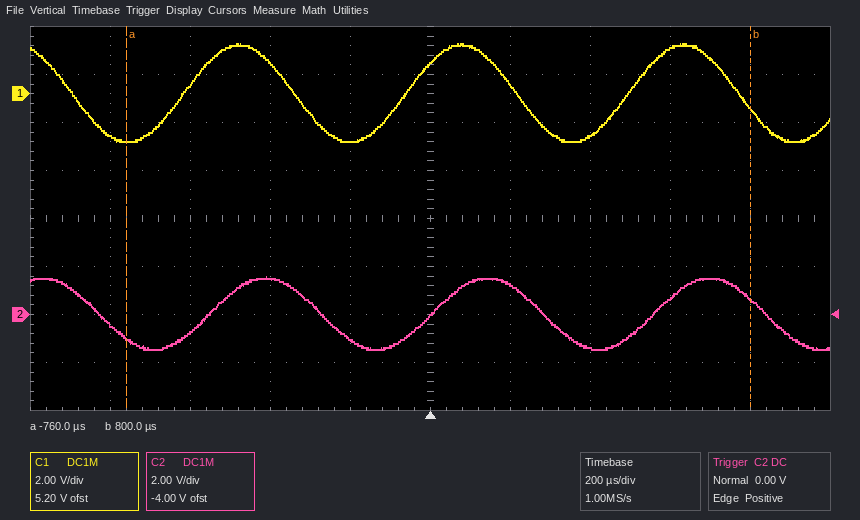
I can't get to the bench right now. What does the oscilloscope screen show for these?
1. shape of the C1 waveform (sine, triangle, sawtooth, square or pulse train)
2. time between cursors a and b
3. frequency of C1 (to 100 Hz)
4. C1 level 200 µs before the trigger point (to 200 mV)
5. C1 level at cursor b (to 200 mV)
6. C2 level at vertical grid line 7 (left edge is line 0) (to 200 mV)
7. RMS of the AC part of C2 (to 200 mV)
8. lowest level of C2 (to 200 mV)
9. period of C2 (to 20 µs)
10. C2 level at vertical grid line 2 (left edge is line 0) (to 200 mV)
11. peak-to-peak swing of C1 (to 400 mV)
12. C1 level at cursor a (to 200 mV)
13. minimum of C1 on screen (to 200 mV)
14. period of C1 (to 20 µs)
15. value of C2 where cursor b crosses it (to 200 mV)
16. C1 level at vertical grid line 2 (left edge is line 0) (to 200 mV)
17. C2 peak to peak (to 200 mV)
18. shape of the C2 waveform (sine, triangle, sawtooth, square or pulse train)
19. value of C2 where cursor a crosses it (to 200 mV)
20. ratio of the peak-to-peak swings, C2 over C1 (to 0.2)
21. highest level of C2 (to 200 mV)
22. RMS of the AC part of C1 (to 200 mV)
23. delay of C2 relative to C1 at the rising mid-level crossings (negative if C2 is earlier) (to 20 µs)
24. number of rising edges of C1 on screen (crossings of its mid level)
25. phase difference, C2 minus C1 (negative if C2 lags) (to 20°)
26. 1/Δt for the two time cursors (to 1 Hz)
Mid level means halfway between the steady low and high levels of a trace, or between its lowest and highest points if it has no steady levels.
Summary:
sine
1.56 ms
1.8 kHz
-2.0 V
-600 mV
-1.4 V
1.0 V
-1.4 V
560 µs
-800 mV
4.0 V
-2.0 V
-2.0 V
560 µs
600 mV
400 mV
3.0 V
sine
-1.0 V
0.8
1.6 V
1.4 V
+60 µs
3
-40°
641 Hz
